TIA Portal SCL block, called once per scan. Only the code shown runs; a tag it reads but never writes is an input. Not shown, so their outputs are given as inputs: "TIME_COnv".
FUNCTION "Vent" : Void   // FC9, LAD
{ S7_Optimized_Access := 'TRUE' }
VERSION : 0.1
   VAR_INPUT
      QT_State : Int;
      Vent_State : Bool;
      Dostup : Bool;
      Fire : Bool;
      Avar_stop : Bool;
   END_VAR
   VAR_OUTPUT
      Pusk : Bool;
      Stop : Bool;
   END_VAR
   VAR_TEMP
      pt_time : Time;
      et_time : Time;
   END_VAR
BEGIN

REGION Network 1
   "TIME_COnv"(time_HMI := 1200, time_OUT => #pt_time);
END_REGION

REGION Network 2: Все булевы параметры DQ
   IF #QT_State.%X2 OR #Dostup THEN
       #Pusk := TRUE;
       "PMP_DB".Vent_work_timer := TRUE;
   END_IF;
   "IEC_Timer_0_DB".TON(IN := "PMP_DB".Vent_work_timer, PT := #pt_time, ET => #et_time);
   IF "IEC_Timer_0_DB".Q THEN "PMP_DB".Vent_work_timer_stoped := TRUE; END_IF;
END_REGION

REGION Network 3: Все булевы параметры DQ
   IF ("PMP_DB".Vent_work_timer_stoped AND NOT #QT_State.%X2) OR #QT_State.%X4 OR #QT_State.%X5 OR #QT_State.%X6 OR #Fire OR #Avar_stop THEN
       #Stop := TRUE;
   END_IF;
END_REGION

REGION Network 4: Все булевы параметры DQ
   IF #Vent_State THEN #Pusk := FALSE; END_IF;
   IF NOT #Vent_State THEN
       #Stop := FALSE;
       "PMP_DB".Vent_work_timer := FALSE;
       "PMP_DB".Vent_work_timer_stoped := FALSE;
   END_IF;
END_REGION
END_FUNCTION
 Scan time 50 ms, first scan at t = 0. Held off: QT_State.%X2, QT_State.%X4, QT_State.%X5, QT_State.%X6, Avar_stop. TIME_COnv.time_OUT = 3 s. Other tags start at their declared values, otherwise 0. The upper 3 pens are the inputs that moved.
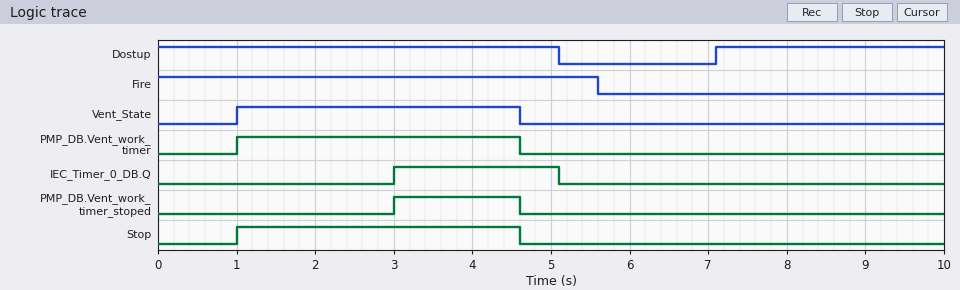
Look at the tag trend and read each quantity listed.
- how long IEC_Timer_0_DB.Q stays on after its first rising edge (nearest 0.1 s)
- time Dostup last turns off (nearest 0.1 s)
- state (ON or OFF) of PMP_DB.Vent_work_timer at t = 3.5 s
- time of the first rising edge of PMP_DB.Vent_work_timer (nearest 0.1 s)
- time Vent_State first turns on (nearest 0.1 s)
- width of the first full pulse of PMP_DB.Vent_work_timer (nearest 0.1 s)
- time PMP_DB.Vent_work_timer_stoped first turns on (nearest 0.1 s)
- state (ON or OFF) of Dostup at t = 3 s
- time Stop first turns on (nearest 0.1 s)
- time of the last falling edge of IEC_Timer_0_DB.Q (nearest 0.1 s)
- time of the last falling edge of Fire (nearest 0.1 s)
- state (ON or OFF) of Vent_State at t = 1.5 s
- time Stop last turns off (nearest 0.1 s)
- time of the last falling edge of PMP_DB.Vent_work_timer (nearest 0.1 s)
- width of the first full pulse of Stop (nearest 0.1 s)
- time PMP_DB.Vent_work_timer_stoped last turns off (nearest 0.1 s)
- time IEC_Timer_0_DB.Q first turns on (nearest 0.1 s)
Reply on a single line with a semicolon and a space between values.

2.1 s; 5.1 s; ON; 1.0 s; 1.0 s; 3.6 s; 3.0 s; ON; 1.0 s; 5.1 s; 5.6 s; ON; 4.6 s; 4.6 s; 3.6 s; 4.6 s; 3.0 s
